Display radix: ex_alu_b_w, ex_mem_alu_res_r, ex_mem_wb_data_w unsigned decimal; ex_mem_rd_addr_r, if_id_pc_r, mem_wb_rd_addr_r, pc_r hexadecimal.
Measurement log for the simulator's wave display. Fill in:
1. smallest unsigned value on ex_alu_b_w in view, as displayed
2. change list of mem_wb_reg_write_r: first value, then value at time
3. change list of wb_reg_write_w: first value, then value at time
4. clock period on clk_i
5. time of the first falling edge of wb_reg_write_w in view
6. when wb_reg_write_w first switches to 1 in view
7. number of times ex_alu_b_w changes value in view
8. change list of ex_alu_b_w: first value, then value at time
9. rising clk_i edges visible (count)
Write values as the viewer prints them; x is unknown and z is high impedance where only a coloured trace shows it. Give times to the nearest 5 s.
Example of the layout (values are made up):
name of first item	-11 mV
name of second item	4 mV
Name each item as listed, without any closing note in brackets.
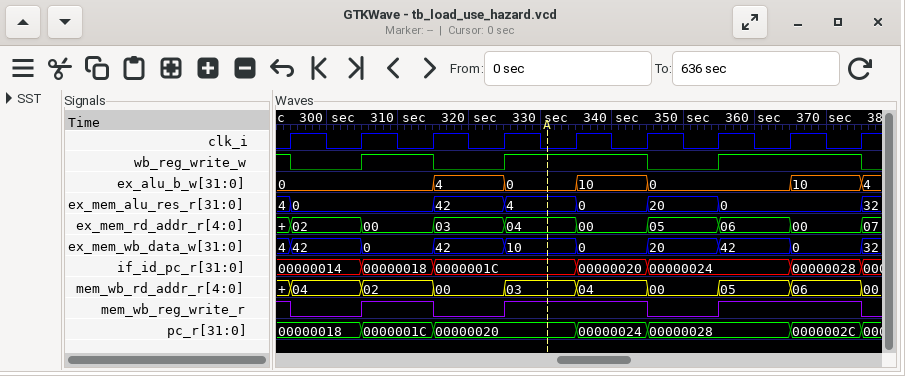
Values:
smallest unsigned value on ex_alu_b_w in view, as displayed	0
change list of mem_wb_reg_write_r: first value, then value at time	1, 0 at 295 s, 1 at 305 s, 0 at 315 s, 1 at 325 s, 0 at 345 s, 1 at 355 s, 0 at 375 s
change list of wb_reg_write_w: first value, then value at time	1, 0 at 295 s, 1 at 305 s, 0 at 315 s, 1 at 325 s, 0 at 345 s, 1 at 355 s, 0 at 375 s
clock period on clk_i	10 s
time of the first falling edge of wb_reg_write_w in view	295 s
when wb_reg_write_w first switches to 1 in view	305 s
number of times ex_alu_b_w changes value in view	6
change list of ex_alu_b_w: first value, then value at time	0, 4 at 315 s, 0 at 325 s, 10 at 335 s, 0 at 345 s, 10 at 365 s, 4 at 375 s
rising clk_i edges visible	9
